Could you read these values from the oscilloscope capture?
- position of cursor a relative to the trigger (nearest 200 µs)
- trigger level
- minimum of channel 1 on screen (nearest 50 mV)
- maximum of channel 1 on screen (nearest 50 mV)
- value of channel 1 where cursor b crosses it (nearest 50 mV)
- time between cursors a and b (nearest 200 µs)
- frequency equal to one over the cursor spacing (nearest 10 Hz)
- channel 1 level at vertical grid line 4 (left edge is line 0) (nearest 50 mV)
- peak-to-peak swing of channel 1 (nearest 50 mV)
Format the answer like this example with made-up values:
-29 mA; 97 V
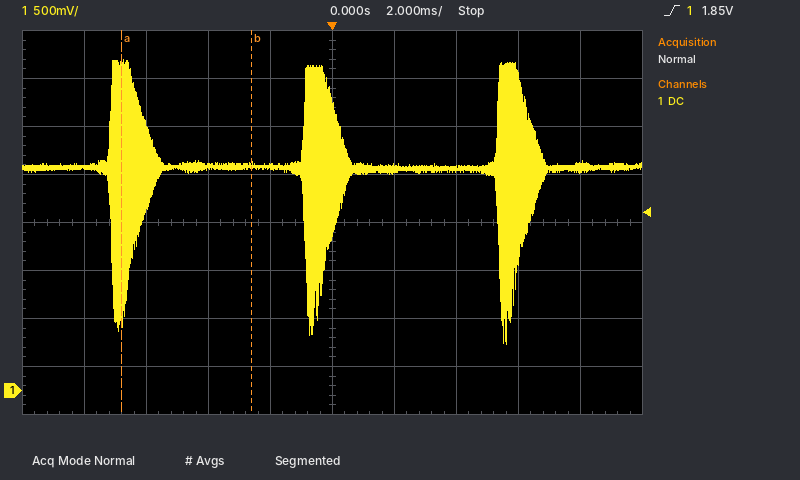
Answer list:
-6.8 ms; 1.85 V; 500 mV; 3.45 V; 2.35 V; 4.2 ms; 240 Hz; 2.35 V; 2.95 V
